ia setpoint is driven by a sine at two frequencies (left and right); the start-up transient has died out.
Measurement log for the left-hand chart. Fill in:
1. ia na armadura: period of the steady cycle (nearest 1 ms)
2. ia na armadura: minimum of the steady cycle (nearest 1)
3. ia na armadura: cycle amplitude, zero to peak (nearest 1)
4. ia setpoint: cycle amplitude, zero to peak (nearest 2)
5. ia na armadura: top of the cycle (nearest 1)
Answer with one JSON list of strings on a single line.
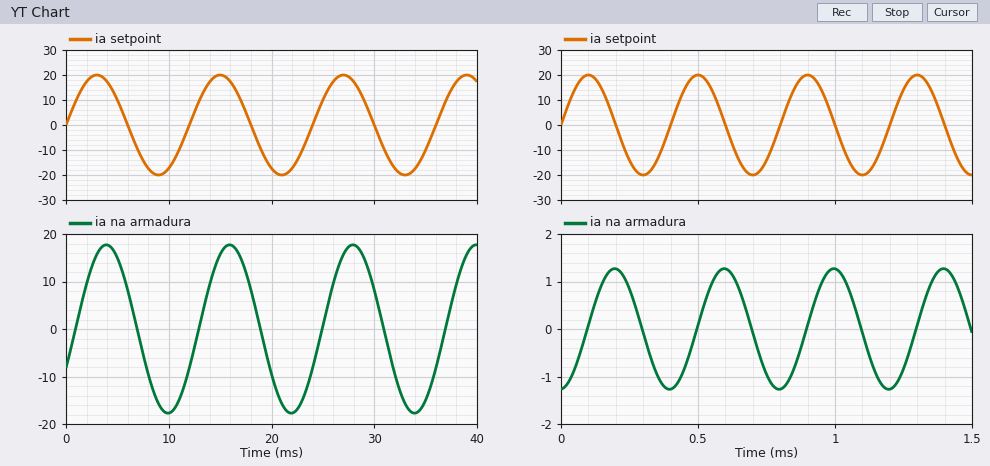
["12 ms", "-18", "18", "20", "18"]
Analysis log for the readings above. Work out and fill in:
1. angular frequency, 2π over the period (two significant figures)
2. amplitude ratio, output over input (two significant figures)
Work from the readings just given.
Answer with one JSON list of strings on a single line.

["0.52 rad/ms", "0.90"]
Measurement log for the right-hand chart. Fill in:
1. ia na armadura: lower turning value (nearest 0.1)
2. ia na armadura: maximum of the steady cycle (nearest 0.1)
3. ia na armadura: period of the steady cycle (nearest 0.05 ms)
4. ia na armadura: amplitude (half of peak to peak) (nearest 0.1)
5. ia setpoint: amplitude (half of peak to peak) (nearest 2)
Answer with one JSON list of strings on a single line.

["-1.3", "1.3", "0.40 ms", "1.3", "20"]
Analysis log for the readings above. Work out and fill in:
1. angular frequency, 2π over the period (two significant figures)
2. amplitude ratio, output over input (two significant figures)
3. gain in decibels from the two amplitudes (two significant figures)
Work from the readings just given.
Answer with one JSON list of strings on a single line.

["16 rad/ms", "0.065", "-24 dB"]
